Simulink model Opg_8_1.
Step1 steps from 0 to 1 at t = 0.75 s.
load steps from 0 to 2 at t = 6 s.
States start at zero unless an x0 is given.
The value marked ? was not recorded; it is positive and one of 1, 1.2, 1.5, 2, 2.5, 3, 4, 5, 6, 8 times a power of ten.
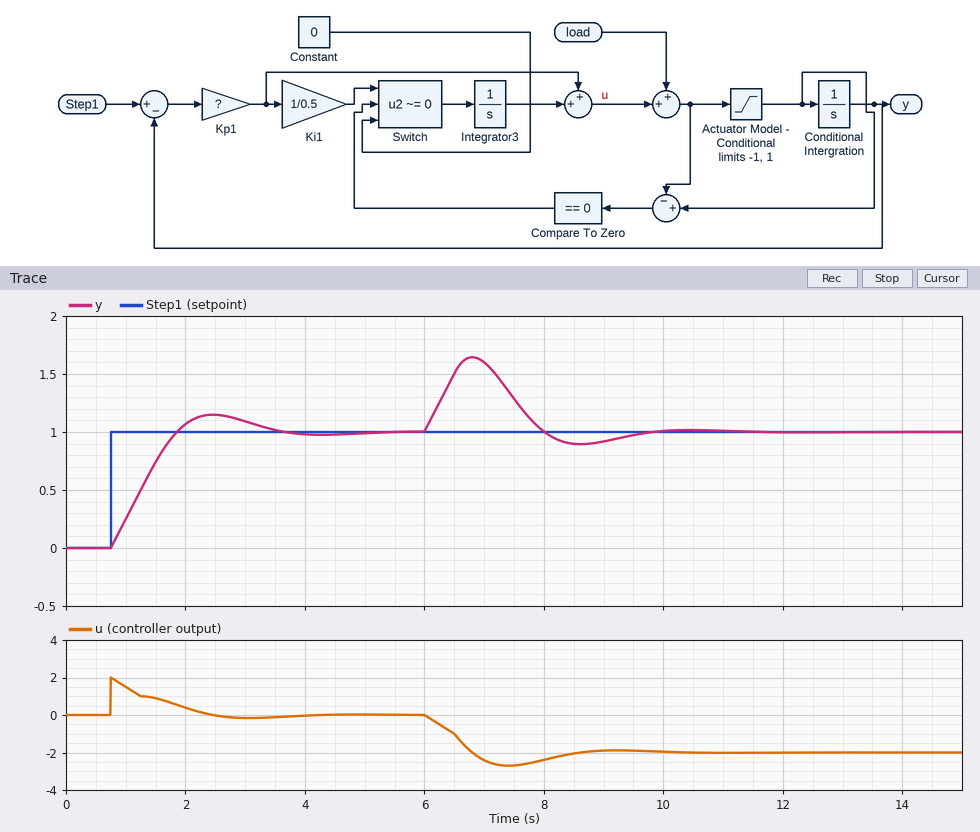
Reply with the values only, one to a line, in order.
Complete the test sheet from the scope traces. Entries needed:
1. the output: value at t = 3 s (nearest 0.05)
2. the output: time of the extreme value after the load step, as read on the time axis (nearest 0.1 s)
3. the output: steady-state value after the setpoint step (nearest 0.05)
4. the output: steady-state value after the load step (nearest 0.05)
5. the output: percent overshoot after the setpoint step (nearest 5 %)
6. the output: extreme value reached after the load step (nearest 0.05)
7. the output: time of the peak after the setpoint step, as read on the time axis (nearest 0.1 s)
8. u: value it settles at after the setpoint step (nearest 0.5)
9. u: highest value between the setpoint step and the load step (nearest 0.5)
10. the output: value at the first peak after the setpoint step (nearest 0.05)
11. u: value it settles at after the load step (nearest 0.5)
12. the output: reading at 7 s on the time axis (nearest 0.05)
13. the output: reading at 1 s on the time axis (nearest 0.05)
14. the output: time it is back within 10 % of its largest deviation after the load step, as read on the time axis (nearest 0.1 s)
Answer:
1.10
6.8 s
1.00
1.00
15 %
1.65
2.5 s
0.0
2.0
1.15
-2.0
1.60
0.25
9.2 s
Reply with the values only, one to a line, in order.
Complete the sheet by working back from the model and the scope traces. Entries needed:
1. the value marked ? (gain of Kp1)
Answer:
2
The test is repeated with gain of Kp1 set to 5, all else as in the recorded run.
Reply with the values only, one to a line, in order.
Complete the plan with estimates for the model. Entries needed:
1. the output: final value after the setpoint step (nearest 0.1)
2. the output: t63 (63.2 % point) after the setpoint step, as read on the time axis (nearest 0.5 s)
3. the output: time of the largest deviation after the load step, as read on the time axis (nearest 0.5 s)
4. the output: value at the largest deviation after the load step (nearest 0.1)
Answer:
1.0
1.5 s
6.5 s
1.3
